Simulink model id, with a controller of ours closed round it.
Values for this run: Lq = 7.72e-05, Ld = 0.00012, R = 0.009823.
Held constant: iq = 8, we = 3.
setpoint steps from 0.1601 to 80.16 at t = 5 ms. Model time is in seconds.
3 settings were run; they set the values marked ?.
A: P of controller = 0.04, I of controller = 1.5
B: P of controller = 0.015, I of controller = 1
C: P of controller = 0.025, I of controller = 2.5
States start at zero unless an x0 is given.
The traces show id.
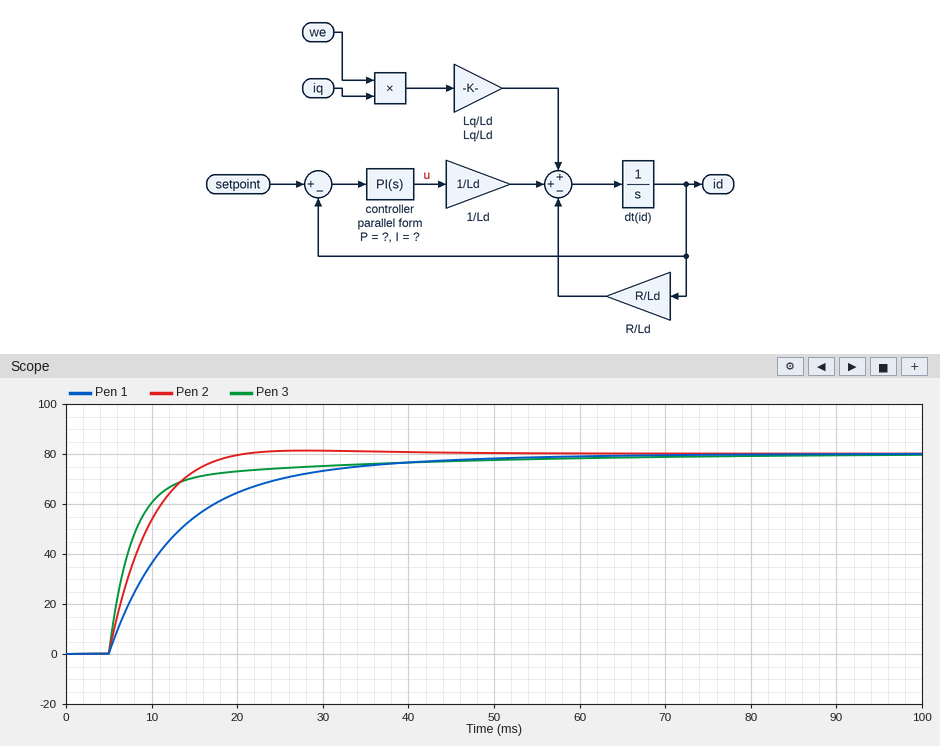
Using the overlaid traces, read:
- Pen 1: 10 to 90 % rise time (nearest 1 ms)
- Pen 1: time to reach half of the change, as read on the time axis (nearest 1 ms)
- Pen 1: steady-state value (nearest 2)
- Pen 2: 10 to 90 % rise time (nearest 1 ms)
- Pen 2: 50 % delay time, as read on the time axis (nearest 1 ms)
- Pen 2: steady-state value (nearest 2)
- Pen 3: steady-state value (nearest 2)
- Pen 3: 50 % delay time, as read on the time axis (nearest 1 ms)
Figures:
22 ms
11 ms
80
9 ms
8 ms
80
80
7 ms
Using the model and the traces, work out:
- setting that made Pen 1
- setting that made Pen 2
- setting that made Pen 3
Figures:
B
C
A
